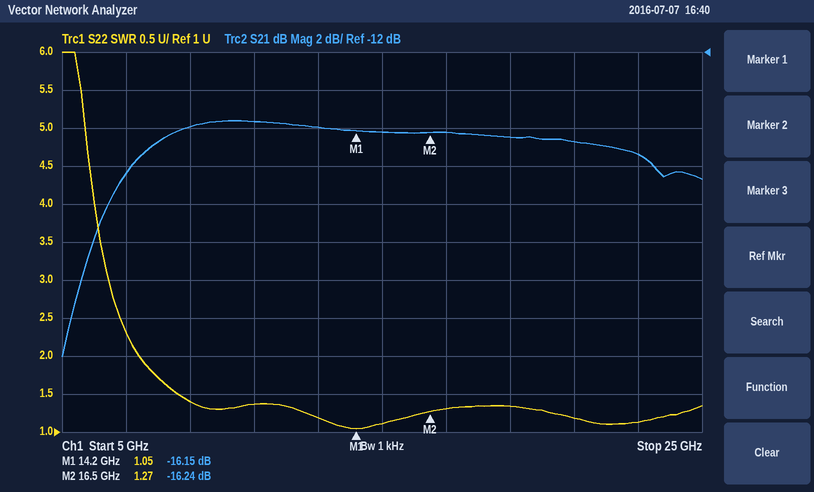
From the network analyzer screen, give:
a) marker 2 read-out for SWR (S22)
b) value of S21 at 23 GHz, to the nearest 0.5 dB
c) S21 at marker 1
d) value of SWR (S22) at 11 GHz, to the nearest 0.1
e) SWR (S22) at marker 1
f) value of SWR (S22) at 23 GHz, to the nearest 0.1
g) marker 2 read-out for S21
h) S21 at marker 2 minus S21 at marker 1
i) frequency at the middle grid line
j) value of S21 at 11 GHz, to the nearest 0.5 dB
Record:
1.27
-17.5 dB
-16.15 dB
1.4
1.05
1.1
-16.24 dB
-0.09 dB
15 GHz
-15.5 dB
